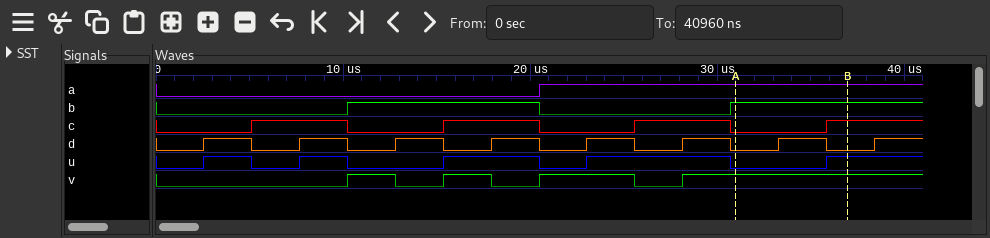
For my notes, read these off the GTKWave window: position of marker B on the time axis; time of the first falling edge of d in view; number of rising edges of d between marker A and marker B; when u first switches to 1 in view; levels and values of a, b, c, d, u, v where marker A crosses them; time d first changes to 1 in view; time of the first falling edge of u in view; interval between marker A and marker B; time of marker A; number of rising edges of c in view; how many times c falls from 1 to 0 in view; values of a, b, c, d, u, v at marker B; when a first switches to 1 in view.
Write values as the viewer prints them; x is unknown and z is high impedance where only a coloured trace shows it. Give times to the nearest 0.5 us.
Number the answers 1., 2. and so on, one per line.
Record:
1. 37 us
2. 5 us
3. 1
4. 2.5 us
5. a=1, b=1, c=0, d=0, u=0, v=1
6. 2.5 us
7. 5 us
8. 6 us
9. 31 us
10. 4
11. 3
12. a=1, b=1, c=1, d=0, u=1, v=1
13. 20.5 us
